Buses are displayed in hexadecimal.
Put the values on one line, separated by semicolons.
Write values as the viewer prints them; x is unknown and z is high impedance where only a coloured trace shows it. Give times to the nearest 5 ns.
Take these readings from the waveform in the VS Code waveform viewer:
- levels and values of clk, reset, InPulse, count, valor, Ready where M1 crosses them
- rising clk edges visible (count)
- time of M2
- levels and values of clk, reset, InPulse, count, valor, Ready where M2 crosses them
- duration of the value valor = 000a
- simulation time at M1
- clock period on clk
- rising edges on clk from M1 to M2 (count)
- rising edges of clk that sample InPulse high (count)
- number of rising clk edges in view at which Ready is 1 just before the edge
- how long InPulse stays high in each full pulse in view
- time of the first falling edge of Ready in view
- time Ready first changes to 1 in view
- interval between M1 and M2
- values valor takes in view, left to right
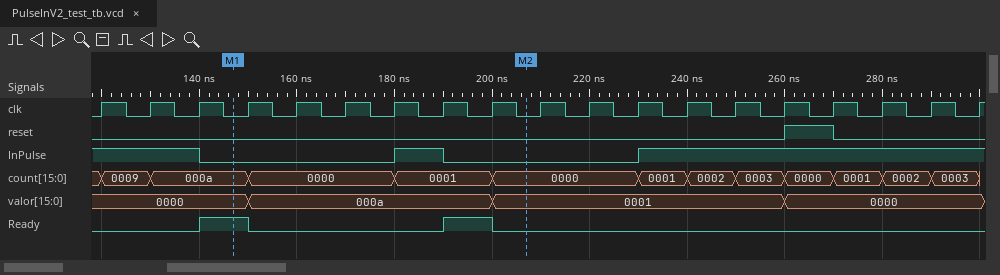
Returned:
clk=0, reset=0, InPulse=0, count=000a, valor=0000, Ready=1; 19; 205 ns; clk=0, reset=0, InPulse=0, count=0000, valor=0001, Ready=0; 50 ns; 145 ns; 10 ns; 6; 11; 2; 10 ns; 150 ns; 140 ns; 60 ns; 0000, 000a, 0001, 0000
